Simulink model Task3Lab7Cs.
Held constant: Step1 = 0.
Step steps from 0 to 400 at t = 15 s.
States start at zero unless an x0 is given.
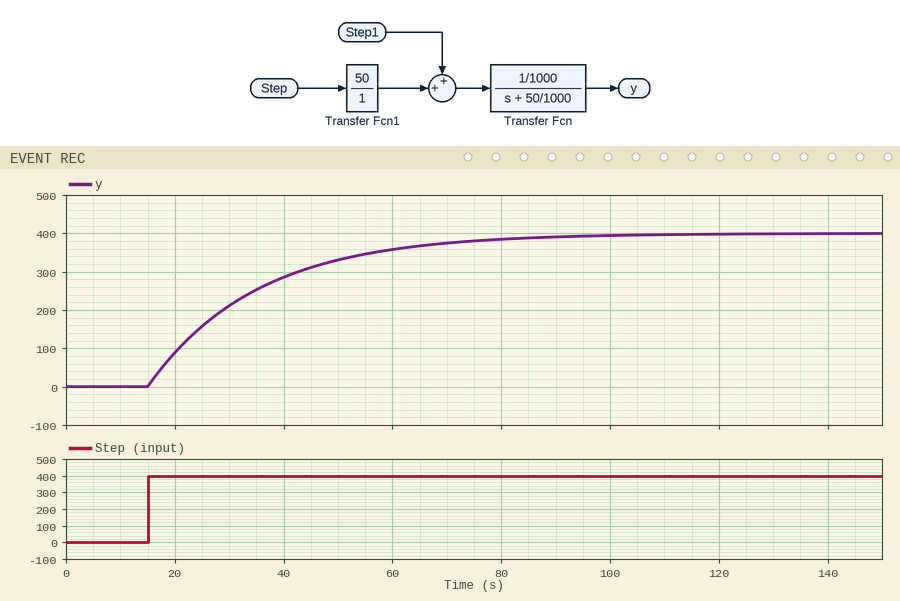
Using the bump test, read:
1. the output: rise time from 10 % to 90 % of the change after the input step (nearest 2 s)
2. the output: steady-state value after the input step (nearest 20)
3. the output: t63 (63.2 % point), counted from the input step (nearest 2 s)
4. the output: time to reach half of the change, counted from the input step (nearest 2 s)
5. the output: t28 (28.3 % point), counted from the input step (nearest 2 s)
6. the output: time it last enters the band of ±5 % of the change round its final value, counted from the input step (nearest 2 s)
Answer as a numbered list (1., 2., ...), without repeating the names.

1. 44 s
2. 400
3. 20 s
4. 14 s
5. 6 s
6. 60 s
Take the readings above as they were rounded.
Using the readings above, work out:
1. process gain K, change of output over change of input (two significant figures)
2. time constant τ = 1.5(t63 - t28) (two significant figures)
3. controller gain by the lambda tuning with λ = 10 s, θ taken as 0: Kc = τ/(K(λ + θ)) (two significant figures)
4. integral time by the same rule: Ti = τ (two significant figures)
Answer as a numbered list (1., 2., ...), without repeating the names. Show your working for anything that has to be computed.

1. (400 - 0) / 400 = 1.0
2. 1.5 × (20 - 6) = 21 s
3. 21 / (1 × (10 + 0)) = 2.1
4. 21 s
